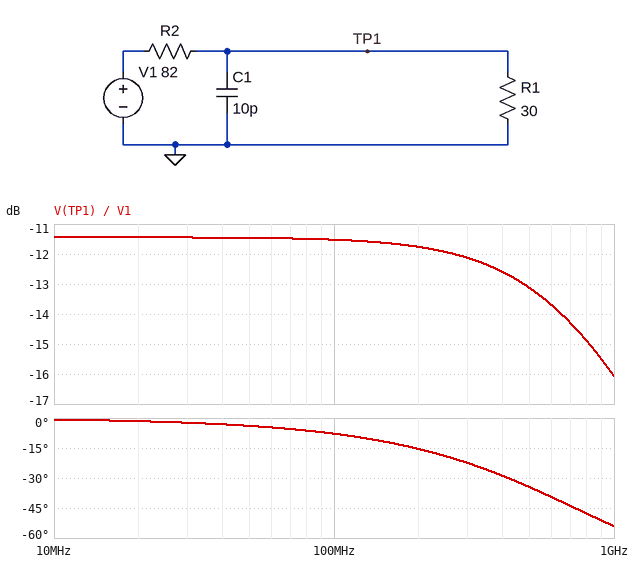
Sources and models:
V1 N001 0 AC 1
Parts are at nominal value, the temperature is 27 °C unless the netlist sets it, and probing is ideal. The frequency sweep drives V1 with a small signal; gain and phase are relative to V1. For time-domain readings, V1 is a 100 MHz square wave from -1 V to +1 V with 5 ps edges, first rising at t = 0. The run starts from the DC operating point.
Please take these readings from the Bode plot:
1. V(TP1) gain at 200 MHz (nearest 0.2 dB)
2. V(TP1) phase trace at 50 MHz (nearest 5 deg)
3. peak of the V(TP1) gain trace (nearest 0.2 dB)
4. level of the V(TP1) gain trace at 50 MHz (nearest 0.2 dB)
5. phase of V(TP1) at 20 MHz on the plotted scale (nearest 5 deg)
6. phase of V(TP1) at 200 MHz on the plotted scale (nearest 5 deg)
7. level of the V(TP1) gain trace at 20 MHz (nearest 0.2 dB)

-11.8 dB
-5 deg
-11.4 dB
-11.4 dB
0 deg
-15 deg
-11.4 dB
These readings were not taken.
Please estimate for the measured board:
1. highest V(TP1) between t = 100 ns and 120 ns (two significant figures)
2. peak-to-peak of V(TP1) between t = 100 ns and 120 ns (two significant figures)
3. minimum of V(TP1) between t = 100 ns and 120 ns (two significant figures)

270 mV
540 mV
-270 mV
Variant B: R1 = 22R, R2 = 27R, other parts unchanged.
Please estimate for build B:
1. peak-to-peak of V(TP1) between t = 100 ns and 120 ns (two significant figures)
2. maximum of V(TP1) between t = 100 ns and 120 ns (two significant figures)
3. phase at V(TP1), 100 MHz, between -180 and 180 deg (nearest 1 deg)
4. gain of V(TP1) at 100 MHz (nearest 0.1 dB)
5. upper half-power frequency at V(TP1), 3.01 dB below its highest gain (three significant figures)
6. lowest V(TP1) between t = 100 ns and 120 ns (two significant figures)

900 mV
450 mV
-4 deg
-7.0 dB
1.31 GHz
-450 mV
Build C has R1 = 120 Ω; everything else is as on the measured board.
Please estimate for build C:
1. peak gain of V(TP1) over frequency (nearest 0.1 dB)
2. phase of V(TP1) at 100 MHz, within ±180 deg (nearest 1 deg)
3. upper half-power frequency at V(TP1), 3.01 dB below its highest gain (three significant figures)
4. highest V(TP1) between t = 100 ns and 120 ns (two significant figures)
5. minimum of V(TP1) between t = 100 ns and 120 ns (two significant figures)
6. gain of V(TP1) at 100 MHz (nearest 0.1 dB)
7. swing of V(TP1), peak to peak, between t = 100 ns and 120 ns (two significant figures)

-4.5 dB
-17 deg
327 MHz
590 mV
-590 mV
-4.9 dB
1.2 V
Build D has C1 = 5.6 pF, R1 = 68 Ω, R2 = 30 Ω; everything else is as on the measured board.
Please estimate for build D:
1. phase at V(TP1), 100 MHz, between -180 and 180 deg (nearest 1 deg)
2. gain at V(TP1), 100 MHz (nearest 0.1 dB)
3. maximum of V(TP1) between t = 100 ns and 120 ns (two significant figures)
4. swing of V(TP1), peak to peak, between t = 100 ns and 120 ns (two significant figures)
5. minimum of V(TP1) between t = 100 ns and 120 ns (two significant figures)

-4 deg
-3.2 dB
690 mV
1.4 V
-690 mV
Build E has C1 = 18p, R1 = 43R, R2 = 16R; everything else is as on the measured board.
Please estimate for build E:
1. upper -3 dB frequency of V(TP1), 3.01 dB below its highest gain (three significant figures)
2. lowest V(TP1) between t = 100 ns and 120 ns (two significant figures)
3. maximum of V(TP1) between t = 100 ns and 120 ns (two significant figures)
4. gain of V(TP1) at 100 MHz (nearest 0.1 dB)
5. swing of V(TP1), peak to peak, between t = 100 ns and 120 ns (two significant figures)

758 MHz
-730 mV
730 mV
-2.8 dB
1.5 V
